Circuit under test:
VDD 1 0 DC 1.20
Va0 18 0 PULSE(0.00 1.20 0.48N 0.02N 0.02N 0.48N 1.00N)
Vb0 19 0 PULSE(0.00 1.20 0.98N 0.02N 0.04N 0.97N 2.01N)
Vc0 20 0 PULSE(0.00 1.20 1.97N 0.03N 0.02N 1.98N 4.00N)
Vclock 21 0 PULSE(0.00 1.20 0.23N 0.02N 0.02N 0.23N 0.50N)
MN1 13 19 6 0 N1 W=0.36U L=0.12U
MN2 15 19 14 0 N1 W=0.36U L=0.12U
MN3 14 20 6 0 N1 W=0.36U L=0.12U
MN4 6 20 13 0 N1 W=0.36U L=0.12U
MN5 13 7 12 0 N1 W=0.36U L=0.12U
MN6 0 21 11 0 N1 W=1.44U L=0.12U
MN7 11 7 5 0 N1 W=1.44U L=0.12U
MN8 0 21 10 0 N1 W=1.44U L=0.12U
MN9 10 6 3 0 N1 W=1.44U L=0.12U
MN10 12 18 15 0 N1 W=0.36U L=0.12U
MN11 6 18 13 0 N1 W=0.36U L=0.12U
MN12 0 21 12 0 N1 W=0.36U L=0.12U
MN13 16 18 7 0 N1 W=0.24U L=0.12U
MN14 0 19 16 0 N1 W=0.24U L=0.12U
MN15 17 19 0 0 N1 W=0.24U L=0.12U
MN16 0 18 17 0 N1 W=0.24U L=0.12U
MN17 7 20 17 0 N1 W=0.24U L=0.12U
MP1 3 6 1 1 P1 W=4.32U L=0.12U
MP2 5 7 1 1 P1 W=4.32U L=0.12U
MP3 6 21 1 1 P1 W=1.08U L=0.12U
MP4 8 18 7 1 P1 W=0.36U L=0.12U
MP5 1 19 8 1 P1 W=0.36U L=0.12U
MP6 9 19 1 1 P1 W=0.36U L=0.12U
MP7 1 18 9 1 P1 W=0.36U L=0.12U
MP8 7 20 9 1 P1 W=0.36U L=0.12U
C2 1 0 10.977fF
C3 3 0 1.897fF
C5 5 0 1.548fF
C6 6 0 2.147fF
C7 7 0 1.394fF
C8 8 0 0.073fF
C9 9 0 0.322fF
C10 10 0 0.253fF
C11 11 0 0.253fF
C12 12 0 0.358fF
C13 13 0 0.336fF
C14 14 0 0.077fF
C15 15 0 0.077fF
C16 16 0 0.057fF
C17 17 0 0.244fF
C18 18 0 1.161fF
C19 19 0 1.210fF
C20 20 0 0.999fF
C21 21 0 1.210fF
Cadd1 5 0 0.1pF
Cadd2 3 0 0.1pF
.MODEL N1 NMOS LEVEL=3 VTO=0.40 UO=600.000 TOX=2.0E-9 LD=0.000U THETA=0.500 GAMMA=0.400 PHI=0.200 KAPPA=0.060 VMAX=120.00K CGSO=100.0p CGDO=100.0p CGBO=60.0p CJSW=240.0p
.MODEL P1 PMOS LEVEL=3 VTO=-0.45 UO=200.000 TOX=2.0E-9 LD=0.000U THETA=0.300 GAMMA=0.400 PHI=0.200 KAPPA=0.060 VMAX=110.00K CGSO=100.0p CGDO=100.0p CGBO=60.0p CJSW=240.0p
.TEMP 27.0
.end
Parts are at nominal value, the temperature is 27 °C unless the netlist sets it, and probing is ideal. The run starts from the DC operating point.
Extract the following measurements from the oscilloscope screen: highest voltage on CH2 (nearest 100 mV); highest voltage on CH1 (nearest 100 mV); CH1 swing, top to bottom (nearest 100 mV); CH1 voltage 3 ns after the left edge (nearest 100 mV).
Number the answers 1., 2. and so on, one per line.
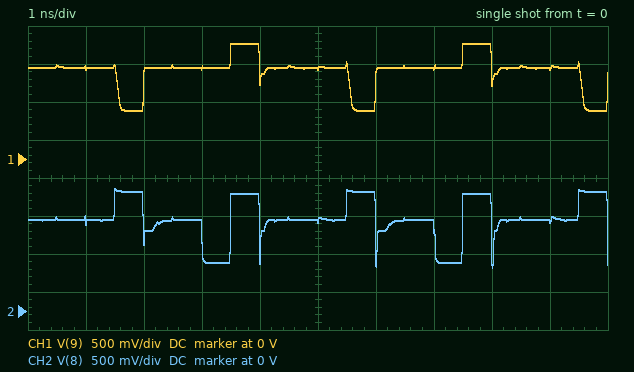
1. 1.6 V
2. 1.5 V
3. 900 mV
4. 1.2 V
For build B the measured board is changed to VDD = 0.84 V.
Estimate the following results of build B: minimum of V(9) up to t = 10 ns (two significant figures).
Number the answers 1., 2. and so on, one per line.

1. 550 mV
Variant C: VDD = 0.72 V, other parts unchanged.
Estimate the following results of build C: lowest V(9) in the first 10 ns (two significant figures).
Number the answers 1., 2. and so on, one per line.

1. 530 mV
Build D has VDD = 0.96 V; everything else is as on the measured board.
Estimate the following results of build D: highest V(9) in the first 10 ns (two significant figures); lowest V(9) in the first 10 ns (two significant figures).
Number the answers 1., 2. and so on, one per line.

1. 1.4 V
2. 580 mV
